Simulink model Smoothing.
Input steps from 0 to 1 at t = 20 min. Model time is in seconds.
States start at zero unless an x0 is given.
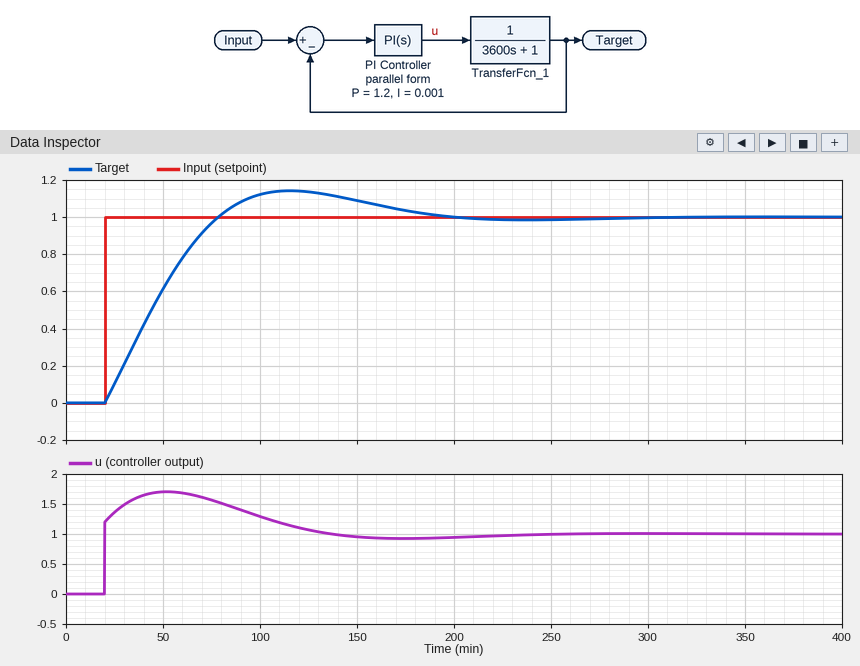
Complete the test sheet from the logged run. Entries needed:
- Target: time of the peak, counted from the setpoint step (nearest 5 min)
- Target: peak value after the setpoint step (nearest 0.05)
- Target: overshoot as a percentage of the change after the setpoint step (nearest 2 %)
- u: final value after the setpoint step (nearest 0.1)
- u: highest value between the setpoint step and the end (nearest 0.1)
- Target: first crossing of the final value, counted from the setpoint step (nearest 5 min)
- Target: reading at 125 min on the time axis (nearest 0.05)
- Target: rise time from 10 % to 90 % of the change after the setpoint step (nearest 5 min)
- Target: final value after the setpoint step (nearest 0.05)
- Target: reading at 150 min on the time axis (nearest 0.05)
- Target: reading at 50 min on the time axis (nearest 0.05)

95 min
1.15
14 %
1.0
1.7
60 min
1.15
45 min
1.00
1.10
0.60
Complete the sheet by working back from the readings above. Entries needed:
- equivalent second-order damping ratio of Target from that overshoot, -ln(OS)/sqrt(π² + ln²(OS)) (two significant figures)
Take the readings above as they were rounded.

0.53
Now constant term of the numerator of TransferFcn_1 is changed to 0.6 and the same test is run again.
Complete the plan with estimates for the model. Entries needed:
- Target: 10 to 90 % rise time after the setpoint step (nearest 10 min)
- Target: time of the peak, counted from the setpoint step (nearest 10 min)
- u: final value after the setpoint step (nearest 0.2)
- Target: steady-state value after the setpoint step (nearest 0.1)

60 min
130 min
1.6
1.0
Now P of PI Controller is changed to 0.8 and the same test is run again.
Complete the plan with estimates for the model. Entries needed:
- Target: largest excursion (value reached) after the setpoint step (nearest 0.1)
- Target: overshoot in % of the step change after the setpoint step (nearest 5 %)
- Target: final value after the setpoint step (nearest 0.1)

1.2
20 %
1.0
